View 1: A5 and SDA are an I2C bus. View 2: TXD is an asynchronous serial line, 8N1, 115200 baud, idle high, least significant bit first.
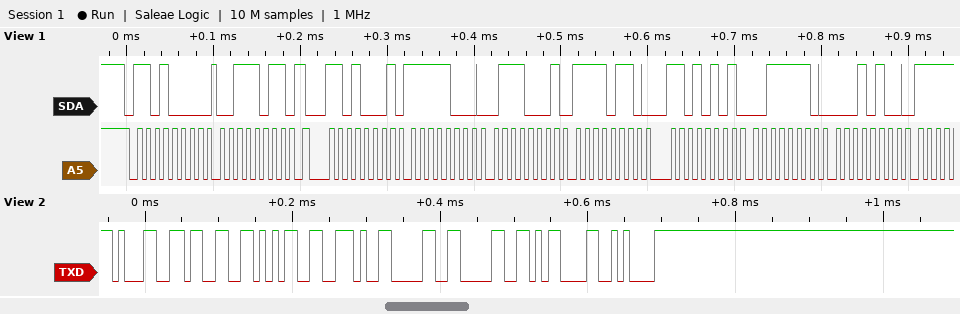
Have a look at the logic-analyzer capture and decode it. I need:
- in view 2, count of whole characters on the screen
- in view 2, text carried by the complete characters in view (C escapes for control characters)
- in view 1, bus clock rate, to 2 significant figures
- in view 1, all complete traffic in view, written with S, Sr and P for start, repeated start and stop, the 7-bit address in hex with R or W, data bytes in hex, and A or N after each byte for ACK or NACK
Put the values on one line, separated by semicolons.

8; "135.00\r\n"; 100 kHz; S 68W A 3B A Sr 68R A F8 A 71 A F6 A D5 A 3E A 14 A
